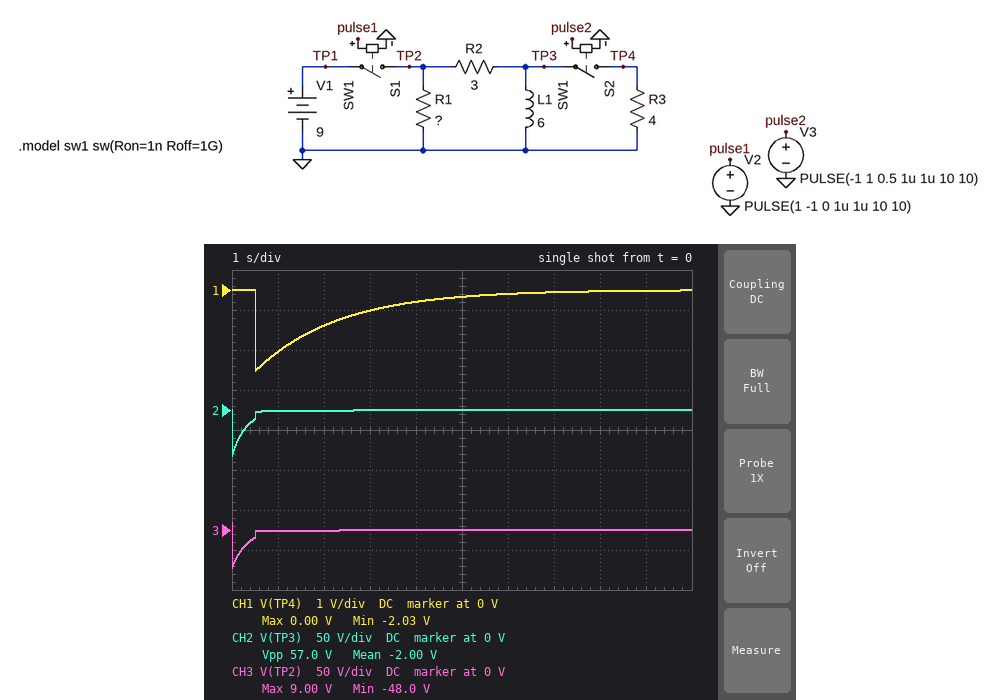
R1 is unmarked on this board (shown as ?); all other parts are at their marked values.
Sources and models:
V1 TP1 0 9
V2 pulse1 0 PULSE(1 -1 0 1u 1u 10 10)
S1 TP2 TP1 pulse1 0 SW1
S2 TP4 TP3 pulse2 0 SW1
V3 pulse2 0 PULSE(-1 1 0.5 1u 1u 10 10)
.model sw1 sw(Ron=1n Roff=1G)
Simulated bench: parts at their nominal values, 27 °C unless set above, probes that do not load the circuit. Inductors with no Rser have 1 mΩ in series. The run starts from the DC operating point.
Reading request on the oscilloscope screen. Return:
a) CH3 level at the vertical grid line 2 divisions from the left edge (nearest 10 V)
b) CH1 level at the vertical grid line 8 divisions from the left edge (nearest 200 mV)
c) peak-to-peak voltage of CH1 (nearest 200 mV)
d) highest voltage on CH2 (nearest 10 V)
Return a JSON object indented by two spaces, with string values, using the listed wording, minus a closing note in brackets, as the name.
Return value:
{
  "CH3 level at the vertical grid line 2 divisions from the left edge": "0 V",
  "CH1 level at the vertical grid line 8 divisions from the left edge": "0 V",
  "peak-to-peak voltage of CH1": "2.0 V",
  "highest voltage on CH2": "0 V"
}
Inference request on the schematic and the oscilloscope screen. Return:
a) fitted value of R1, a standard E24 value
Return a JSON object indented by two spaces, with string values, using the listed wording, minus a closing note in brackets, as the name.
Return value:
{
  "fitted value of R1, a standard E24 value": "16 Ω"
}
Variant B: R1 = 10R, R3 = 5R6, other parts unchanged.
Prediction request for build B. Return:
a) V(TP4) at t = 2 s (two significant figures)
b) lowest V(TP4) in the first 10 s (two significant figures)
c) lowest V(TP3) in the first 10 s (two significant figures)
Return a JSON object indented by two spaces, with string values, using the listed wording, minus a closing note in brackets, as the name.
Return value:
{
  "V(TP4) at t = 2 s": "-1.5 V",
  "lowest V(TP4) in the first 10 s": "-4.0 V",
  "lowest V(TP3) in the first 10 s": "-39 V"
}
